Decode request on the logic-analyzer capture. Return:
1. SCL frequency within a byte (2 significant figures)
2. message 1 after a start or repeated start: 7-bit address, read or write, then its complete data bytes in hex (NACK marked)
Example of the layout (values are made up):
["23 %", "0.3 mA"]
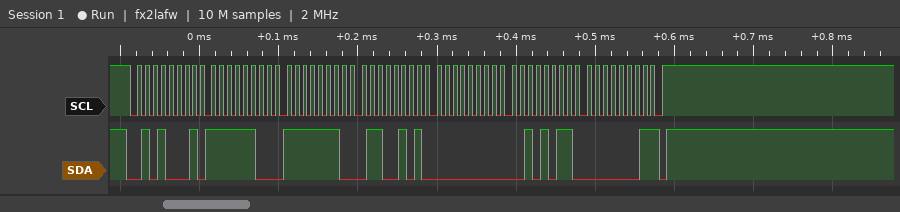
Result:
["100 kHz", "0x28 read: FC FE 65 00 2B 01 NACK"]
